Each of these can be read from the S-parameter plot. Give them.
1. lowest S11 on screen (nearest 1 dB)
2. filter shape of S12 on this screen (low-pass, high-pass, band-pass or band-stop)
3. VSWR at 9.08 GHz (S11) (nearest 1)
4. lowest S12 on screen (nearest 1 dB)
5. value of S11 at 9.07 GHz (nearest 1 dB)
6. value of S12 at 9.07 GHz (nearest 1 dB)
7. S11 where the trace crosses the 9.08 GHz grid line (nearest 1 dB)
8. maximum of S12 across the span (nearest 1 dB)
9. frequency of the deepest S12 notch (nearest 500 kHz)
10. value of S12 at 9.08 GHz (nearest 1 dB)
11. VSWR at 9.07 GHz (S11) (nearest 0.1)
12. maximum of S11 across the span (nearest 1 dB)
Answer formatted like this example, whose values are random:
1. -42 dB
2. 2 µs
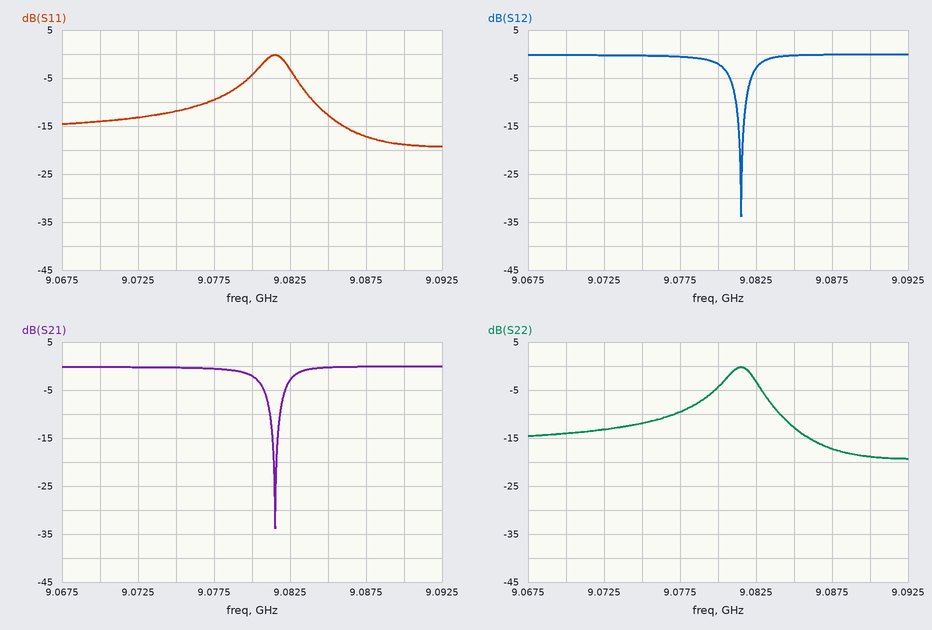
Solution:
1. -19 dB
2. band-stop
3. 4
4. -34 dB
5. -14 dB
6. 0 dB
7. -4 dB
8. 0 dB
9. 9.0815 GHz
10. -2 dB
11. 1.5
12. 0 dB
